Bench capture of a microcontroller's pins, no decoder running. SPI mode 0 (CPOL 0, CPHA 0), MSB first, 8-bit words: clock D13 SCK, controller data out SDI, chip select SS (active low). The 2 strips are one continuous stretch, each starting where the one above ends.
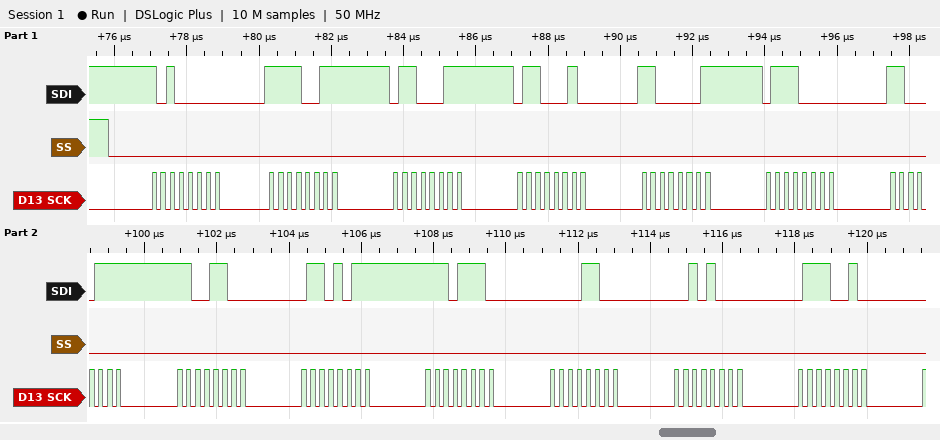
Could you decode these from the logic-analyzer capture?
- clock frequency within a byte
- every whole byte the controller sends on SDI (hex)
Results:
4 MHz
0xA0 0xF3 0x63 0x62 0xC1 0x70 0xC7 0xCC 0x6B 0xEE 0x0C 0x28 0x72
